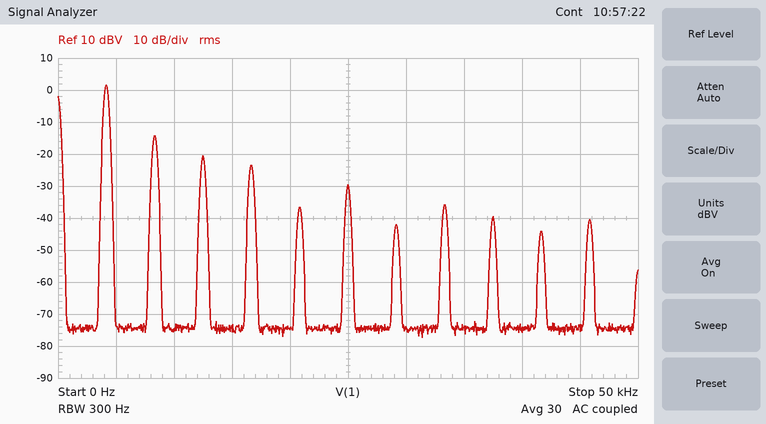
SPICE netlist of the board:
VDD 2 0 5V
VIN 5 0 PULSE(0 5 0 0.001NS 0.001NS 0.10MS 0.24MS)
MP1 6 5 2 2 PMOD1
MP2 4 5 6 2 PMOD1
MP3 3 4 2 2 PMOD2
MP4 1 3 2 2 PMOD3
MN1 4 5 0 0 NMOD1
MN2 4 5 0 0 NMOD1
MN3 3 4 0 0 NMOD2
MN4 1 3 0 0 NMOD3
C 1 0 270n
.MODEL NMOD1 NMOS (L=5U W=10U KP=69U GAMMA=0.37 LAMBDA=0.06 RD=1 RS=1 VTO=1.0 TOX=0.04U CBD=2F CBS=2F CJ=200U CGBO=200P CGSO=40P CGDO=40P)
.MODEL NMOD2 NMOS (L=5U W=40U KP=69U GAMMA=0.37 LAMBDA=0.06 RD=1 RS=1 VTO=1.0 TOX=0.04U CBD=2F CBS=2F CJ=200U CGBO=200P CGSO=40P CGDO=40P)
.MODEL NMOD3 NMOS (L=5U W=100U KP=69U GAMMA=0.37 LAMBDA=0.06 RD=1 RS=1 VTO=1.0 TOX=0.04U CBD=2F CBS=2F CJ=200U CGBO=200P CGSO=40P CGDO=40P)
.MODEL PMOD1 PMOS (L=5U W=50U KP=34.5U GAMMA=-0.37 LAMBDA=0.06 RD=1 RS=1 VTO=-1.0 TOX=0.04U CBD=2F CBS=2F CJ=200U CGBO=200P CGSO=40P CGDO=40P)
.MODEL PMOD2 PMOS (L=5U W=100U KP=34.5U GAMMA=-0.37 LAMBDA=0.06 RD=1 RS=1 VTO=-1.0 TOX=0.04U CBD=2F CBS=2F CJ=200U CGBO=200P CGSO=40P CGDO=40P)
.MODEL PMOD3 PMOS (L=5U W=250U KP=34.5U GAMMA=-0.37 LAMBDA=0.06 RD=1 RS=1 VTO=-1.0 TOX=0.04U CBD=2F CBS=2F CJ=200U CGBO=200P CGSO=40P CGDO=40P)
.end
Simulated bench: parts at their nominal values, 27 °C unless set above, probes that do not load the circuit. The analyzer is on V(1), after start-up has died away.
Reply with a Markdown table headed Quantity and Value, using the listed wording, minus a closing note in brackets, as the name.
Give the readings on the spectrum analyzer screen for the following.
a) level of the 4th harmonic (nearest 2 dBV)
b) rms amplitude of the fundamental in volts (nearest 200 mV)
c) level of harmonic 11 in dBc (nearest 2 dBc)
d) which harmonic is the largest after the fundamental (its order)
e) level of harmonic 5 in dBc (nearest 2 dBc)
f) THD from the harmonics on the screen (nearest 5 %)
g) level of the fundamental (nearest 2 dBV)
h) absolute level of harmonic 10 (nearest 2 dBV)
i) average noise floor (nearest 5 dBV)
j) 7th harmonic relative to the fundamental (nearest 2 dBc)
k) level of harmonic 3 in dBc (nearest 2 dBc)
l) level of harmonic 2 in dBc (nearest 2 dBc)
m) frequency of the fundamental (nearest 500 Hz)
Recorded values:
| Quantity | Value |
|---|---|
| level of the 4th harmonic | -24 dBV |
| rms amplitude of the fundamental in volts | 1.2 V |
| level of harmonic 11 in dBc | -42 dBc |
| which harmonic is the largest after the fundamental | 2 |
| level of harmonic 5 in dBc | -38 dBc |
| THD from the harmonics on the screen | 20 % |
| level of the fundamental | 2 dBV |
| absolute level of harmonic 10 | -44 dBV |
| average noise floor | -75 dBV |
| 7th harmonic relative to the fundamental | -44 dBc |
| level of harmonic 3 in dBc | -22 dBc |
| level of harmonic 2 in dBc | -16 dBc |
| frequency of the fundamental | 4.0 kHz |
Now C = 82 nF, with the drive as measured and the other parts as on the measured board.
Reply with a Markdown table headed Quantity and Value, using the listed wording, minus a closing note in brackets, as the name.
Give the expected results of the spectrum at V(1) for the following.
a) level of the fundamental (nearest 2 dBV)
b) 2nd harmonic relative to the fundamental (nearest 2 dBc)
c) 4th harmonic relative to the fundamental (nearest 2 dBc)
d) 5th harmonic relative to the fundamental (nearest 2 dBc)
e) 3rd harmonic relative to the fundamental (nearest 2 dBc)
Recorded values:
| Quantity | Value |
|---|---|
| level of the fundamental | 6 dBV |
| 2nd harmonic relative to the fundamental | -12 dBc |
| 4th harmonic relative to the fundamental | -18 dBc |
| 5th harmonic relative to the fundamental | -34 dBc |
| 3rd harmonic relative to the fundamental | -16 dBc |
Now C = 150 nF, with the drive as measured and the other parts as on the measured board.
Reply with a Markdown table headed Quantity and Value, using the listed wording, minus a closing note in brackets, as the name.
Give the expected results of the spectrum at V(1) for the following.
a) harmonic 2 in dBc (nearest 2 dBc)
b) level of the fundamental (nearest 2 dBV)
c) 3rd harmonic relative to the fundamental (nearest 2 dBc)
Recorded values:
| Quantity | Value |
|---|---|
| harmonic 2 in dBc | -14 dBc |
| level of the fundamental | 4 dBV |
| 3rd harmonic relative to the fundamental | -20 dBc |
